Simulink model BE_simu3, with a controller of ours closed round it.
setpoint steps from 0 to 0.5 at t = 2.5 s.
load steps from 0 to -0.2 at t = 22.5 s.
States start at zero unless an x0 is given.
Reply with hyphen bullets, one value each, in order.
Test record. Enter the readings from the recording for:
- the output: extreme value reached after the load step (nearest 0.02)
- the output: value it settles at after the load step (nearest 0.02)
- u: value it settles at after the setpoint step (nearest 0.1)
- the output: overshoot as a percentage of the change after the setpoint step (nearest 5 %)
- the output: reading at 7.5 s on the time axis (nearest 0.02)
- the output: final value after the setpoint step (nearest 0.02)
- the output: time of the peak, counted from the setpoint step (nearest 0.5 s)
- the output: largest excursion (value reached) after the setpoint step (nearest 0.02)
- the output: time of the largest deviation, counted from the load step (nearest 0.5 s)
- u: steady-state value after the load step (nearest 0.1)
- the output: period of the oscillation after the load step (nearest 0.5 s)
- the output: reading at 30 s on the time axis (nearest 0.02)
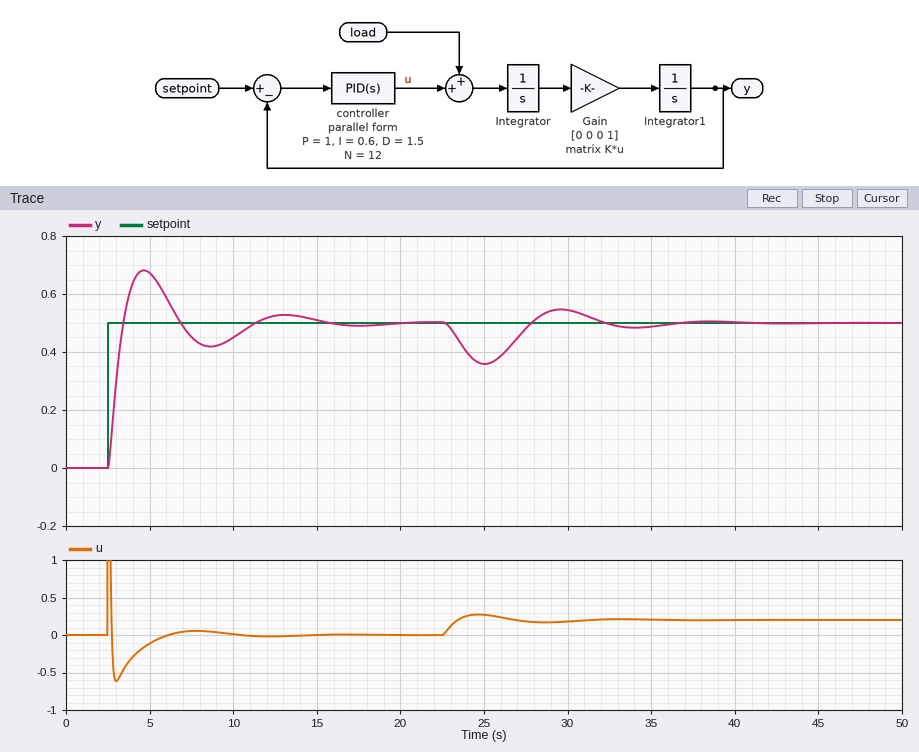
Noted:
- 0.36
- 0.50
- 0.0
- 35 %
- 0.46
- 0.50
- 2.0 s
- 0.68
- 2.5 s
- 0.2
- 9.0 s
- 0.54
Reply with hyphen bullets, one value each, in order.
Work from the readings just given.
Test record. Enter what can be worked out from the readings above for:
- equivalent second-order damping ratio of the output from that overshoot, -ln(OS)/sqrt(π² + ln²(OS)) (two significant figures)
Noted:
- 0.32
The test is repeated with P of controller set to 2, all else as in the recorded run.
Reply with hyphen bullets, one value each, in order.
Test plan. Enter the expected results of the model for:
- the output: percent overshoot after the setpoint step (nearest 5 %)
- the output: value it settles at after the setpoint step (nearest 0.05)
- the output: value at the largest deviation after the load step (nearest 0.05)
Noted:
- 40 %
- 0.50
- 0.40
